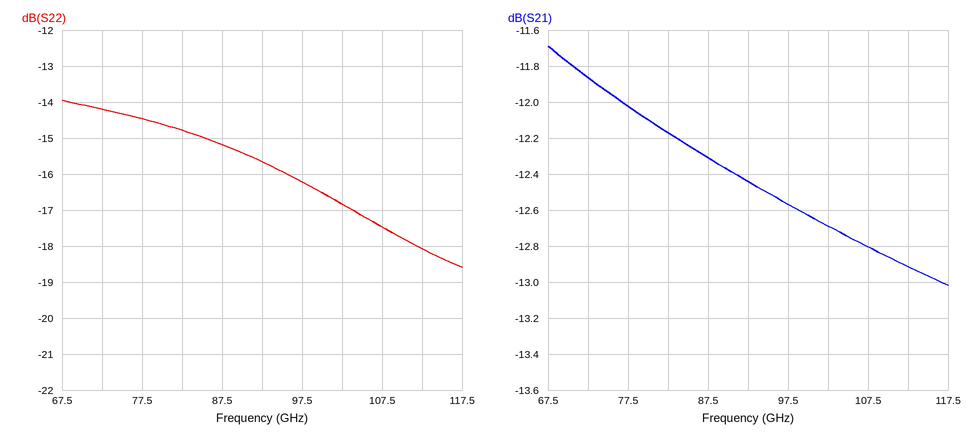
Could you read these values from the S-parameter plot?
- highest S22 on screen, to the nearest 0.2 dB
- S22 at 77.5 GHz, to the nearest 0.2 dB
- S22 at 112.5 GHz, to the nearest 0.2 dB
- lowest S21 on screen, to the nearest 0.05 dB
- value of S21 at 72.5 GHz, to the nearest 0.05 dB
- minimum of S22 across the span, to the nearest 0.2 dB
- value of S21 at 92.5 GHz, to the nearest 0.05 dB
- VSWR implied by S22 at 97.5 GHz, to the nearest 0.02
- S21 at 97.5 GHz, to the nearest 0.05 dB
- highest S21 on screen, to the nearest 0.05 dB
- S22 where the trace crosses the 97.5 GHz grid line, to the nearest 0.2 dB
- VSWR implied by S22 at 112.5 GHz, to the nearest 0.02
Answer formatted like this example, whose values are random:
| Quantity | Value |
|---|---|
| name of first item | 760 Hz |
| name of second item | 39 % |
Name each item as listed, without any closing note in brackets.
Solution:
| Quantity | Value |
|---|---|
| highest S22 on screen, to the nearest 0.2 dB | -14.0 dB |
| S22 at 77.5 GHz, to the nearest 0.2 dB | -14.4 dB |
| S22 at 112.5 GHz, to the nearest 0.2 dB | -18.0 dB |
| lowest S21 on screen, to the nearest 0.05 dB | -13.00 dB |
| value of S21 at 72.5 GHz, to the nearest 0.05 dB | -11.85 dB |
| minimum of S22 across the span, to the nearest 0.2 dB | -18.6 dB |
| value of S21 at 92.5 GHz, to the nearest 0.05 dB | -12.45 dB |
| VSWR implied by S22 at 97.5 GHz, to the nearest 0.02 | 1.36 |
| S21 at 97.5 GHz, to the nearest 0.05 dB | -12.55 dB |
| highest S21 on screen, to the nearest 0.05 dB | -11.70 dB |
| S22 where the trace crosses the 97.5 GHz grid line, to the nearest 0.2 dB | -16.2 dB |
| VSWR implied by S22 at 112.5 GHz, to the nearest 0.02 | 1.28 |
